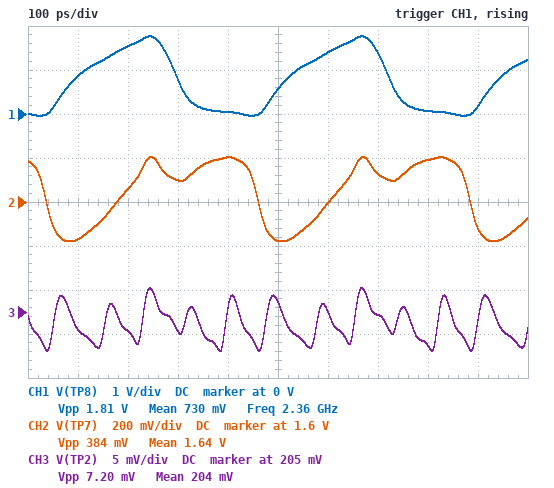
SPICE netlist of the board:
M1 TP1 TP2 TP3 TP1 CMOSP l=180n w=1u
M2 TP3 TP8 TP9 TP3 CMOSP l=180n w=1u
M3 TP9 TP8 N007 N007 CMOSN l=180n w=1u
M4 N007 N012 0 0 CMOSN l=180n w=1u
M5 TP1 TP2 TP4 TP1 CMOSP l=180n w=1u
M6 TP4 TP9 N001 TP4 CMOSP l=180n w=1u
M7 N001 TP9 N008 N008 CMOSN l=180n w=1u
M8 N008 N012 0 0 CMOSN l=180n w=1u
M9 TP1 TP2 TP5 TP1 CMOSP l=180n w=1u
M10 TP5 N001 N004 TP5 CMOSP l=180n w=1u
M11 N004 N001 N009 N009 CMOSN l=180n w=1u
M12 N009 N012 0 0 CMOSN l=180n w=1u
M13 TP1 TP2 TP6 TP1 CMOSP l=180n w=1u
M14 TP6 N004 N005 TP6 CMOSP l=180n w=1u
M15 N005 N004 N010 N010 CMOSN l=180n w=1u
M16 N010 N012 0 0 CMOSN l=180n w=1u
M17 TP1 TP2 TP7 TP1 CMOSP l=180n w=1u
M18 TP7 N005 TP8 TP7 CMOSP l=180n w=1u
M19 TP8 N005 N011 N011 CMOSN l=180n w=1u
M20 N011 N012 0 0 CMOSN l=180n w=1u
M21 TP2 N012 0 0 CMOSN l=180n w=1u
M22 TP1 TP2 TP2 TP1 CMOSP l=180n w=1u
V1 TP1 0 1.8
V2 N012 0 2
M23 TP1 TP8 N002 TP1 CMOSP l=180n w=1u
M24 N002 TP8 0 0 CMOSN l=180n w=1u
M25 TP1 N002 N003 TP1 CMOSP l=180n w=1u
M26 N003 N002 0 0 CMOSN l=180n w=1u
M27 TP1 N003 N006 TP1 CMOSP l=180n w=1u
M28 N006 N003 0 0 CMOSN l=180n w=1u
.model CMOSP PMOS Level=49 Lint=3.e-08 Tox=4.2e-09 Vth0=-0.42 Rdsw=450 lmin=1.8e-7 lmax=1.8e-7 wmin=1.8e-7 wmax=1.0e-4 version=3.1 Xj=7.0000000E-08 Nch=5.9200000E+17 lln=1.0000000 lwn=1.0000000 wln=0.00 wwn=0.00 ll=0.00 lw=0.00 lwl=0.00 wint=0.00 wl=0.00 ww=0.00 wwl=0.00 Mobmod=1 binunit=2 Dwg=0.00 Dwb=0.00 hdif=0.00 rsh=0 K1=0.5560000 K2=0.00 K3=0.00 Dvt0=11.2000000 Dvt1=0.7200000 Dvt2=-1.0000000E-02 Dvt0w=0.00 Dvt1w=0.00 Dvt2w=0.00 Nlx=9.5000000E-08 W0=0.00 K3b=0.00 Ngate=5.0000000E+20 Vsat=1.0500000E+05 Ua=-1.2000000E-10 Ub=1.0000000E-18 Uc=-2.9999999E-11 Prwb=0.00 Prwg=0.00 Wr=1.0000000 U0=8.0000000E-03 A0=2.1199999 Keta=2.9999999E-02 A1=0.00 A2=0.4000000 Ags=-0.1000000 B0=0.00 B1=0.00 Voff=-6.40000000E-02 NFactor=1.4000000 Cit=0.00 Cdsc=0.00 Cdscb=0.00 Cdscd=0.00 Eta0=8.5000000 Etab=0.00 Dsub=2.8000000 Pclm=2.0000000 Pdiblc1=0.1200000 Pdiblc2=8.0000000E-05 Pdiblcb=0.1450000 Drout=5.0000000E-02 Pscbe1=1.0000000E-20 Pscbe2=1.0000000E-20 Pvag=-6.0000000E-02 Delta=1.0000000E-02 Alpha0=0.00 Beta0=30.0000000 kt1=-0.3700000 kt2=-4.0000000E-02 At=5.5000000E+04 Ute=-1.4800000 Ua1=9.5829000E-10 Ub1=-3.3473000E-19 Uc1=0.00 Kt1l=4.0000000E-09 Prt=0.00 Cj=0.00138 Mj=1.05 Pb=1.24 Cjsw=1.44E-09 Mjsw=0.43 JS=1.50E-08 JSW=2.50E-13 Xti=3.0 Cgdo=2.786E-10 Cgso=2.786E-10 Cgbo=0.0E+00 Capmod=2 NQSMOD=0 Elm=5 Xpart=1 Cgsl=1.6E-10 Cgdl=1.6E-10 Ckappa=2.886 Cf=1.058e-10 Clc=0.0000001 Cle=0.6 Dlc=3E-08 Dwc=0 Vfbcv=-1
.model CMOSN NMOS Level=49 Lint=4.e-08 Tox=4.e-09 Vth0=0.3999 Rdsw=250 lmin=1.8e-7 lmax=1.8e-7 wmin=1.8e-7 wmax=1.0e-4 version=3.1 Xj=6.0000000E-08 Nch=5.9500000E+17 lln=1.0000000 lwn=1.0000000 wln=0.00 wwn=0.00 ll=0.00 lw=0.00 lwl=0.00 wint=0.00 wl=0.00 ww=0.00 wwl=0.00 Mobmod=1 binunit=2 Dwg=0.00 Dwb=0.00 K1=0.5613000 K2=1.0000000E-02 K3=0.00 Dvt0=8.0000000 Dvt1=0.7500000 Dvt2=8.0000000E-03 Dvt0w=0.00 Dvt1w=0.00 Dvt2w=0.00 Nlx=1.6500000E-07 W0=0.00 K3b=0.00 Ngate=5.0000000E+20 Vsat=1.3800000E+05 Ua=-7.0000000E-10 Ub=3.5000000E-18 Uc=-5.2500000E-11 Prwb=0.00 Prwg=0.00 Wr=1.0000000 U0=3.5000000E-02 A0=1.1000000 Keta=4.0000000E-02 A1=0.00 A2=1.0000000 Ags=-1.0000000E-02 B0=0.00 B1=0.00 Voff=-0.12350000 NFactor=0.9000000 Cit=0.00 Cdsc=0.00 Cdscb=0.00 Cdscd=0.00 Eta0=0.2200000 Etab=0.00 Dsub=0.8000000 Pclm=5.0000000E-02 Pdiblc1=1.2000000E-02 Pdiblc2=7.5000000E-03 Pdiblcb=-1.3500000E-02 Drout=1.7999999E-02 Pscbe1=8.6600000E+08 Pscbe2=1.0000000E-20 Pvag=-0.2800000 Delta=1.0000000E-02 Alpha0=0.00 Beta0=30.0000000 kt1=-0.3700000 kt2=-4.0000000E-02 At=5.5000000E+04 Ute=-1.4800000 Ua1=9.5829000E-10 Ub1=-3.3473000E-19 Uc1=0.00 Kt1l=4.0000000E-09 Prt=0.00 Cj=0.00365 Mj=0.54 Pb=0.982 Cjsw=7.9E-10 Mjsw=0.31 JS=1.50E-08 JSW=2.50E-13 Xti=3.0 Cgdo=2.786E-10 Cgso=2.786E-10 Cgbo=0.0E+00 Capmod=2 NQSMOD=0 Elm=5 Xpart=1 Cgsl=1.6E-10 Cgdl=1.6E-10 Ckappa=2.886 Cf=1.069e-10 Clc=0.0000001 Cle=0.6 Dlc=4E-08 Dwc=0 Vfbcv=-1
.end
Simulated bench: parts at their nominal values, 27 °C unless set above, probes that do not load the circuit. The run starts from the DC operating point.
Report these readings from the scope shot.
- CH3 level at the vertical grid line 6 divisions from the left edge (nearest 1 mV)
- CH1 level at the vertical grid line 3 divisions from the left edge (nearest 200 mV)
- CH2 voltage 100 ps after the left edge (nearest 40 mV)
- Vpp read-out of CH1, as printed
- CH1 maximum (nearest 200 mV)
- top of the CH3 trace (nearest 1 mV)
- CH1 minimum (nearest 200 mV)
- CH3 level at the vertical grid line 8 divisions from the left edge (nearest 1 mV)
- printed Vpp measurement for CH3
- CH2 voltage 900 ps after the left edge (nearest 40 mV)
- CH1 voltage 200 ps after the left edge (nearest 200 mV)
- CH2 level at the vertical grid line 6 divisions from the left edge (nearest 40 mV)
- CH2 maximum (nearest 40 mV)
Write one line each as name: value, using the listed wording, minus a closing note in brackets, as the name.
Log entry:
CH3 level at the vertical grid line 6 divisions from the left edge: 205 mV
CH1 level at the vertical grid line 3 divisions from the left edge: 800 mV
CH2 voltage 100 ps after the left edge: 1.44 V
Vpp read-out of CH1, as printed: 1.81 V
CH1 maximum: 1.8 V
top of the CH3 trace: 208 mV
CH1 minimum: 0 V
CH3 level at the vertical grid line 8 divisions from the left edge: 201 mV
printed Vpp measurement for CH3: 7.20 mV
CH2 voltage 900 ps after the left edge: 1.48 V
CH1 voltage 200 ps after the left edge: 1.6 V
CH2 level at the vertical grid line 6 divisions from the left edge: 1.60 V
CH2 maximum: 1.80 V
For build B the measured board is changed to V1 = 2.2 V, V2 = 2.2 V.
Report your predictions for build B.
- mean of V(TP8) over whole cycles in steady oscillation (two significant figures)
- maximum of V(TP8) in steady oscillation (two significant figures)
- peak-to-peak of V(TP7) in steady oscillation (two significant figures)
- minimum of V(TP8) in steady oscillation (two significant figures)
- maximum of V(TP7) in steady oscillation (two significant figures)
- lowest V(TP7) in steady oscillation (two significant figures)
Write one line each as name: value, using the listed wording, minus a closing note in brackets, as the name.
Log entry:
mean of V(TP8) over whole cycles in steady oscillation: 920 mV
maximum of V(TP8) in steady oscillation: 2.1 V
peak-to-peak of V(TP7) in steady oscillation: 480 mV
minimum of V(TP8) in steady oscillation: -38 mV
maximum of V(TP7) in steady oscillation: 2.2 V
lowest V(TP7) in steady oscillation: 1.7 V
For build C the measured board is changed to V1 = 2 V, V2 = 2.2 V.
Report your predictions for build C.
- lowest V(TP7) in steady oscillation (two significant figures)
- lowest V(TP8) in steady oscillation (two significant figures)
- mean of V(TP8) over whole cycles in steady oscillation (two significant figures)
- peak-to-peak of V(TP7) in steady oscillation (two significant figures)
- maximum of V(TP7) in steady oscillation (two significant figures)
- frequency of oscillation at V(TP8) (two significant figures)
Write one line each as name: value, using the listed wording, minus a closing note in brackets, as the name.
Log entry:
lowest V(TP7) in steady oscillation: 1.6 V
lowest V(TP8) in steady oscillation: -40 mV
mean of V(TP8) over whole cycles in steady oscillation: 840 mV
peak-to-peak of V(TP7) in steady oscillation: 430 mV
maximum of V(TP7) in steady oscillation: 2.0 V
frequency of oscillation at V(TP8): 2.6 GHz
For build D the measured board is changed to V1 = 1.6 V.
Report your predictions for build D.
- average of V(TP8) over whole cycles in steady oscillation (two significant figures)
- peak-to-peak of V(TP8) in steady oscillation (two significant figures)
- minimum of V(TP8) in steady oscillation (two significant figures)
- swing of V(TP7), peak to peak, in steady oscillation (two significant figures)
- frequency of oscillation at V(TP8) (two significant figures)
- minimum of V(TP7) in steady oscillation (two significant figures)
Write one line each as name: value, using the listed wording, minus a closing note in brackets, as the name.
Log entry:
average of V(TP8) over whole cycles in steady oscillation: 680 mV
peak-to-peak of V(TP8) in steady oscillation: 1.6 V
minimum of V(TP8) in steady oscillation: -41 mV
swing of V(TP7), peak to peak, in steady oscillation: 340 mV
frequency of oscillation at V(TP8): 2.1 GHz
minimum of V(TP7) in steady oscillation: 1.3 V
